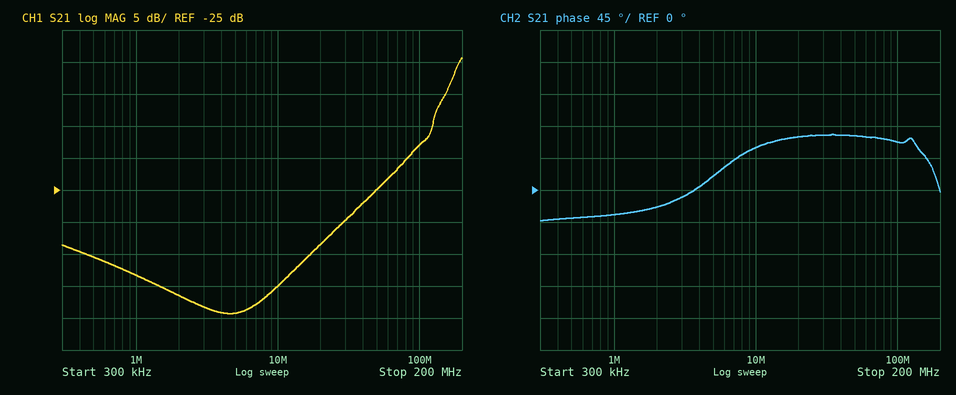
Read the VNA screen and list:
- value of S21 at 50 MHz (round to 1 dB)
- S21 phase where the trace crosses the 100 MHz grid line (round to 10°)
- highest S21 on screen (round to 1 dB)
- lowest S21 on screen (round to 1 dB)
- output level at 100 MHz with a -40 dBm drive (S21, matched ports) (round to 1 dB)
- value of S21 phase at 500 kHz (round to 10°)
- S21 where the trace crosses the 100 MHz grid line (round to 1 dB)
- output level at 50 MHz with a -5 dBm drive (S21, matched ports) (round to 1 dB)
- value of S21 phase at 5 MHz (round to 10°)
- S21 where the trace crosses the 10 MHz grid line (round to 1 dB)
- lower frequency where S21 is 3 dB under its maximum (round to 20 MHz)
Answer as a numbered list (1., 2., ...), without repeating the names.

1. -25 dB
2. 70°
3. -4 dB
4. -44 dB
5. -58 dBm
6. -40°
7. -18 dB
8. -30 dBm
9. 20°
10. -40 dB
11. 180 MHz
